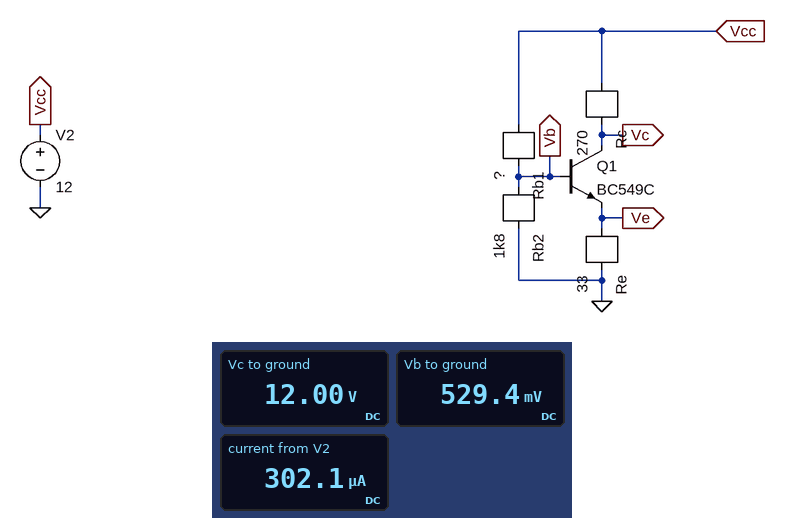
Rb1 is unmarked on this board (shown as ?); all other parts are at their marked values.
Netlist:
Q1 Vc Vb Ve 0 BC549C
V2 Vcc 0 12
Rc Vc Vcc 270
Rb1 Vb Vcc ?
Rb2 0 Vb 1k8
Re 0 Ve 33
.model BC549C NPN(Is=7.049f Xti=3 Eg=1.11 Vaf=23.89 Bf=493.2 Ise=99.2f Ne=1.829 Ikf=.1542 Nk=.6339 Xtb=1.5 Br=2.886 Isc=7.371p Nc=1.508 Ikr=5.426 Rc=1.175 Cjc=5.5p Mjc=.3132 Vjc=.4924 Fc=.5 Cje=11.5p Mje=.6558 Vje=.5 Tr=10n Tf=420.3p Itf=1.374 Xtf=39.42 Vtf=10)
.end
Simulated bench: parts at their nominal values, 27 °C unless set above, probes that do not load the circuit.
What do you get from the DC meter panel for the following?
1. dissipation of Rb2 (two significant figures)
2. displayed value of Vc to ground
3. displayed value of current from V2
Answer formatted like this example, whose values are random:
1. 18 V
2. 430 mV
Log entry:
1. 160 µW
2. 12.00 V
3. 302.1 µA
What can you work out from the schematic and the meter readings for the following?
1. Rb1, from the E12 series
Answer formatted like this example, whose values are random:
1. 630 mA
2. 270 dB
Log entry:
1. 39 kΩ
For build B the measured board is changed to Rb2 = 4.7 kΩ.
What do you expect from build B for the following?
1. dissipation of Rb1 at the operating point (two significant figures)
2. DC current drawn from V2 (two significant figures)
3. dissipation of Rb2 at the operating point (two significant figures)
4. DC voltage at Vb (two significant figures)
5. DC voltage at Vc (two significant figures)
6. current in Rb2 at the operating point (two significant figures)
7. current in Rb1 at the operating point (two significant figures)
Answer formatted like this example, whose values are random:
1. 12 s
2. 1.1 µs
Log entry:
1. 3.0 mW
2. 14 mA
3. 300 µW
4. 1.2 V
5. 8.2 V
6. 250 µA
7. 280 µA
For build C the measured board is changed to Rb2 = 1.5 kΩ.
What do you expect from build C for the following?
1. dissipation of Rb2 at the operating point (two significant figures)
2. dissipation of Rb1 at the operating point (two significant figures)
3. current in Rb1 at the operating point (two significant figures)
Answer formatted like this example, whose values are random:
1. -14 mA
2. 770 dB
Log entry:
1. 130 µW
2. 3.4 mW
3. 300 µA
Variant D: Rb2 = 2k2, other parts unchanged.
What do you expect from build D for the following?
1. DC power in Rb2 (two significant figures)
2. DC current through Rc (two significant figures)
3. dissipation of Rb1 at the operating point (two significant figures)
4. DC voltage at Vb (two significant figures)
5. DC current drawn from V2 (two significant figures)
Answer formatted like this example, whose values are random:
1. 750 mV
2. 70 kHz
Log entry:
1. 190 µW
2. 360 µA
3. 3.3 mW
4. 640 mV
5. 650 µA
